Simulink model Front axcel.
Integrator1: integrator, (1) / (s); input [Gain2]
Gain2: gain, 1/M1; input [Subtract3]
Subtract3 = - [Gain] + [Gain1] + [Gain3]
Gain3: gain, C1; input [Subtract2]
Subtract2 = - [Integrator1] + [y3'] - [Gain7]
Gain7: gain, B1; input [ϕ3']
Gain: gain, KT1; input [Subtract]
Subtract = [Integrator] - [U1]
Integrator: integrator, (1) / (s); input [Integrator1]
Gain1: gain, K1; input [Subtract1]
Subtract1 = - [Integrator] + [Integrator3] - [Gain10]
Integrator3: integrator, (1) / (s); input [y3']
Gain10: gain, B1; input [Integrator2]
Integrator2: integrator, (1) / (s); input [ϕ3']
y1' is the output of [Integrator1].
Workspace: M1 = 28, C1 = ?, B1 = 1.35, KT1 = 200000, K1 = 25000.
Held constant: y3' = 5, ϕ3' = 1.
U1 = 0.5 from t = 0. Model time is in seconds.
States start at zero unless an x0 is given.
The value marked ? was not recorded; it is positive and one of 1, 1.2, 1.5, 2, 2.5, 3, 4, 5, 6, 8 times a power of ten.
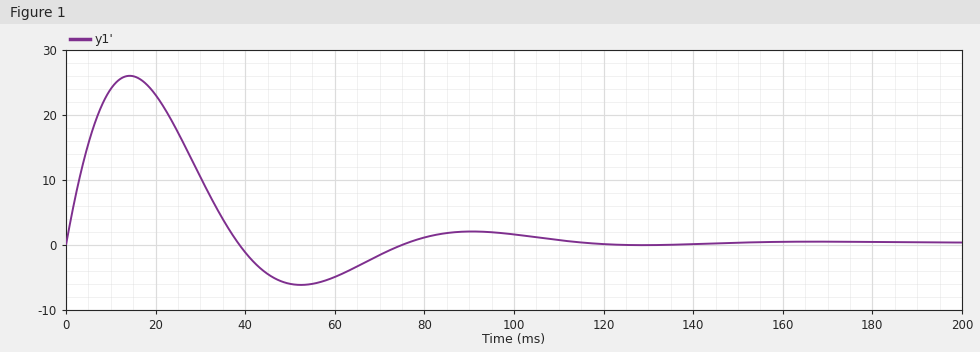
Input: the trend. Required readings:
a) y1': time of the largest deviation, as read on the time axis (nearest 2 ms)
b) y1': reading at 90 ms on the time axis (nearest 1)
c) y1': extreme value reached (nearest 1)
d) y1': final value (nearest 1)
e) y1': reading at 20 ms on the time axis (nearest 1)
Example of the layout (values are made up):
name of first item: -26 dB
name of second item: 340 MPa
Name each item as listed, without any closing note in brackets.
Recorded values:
y1': time of the largest deviation, as read on the time axis: 14 ms
y1': reading at 90 ms on the time axis: 2
y1': extreme value reached: 26
y1': final value: 0
y1': reading at 20 ms on the time axis: 23
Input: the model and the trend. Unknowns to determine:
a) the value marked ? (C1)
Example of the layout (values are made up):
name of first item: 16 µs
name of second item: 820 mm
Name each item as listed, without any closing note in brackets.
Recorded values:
the value marked ?: 2000
